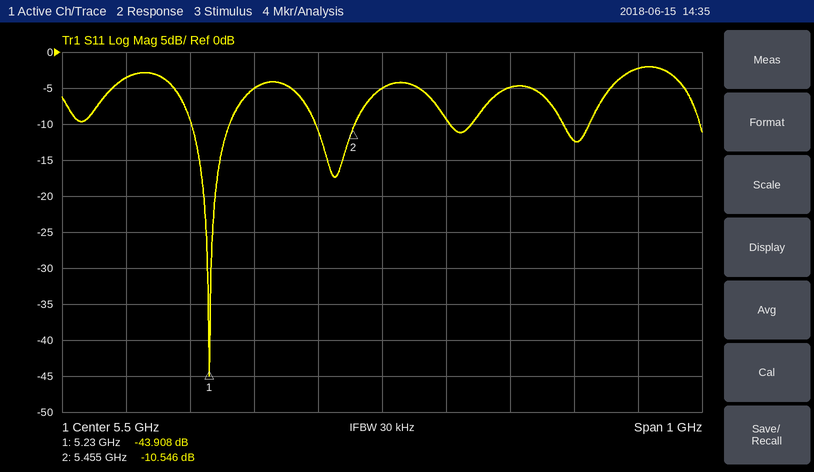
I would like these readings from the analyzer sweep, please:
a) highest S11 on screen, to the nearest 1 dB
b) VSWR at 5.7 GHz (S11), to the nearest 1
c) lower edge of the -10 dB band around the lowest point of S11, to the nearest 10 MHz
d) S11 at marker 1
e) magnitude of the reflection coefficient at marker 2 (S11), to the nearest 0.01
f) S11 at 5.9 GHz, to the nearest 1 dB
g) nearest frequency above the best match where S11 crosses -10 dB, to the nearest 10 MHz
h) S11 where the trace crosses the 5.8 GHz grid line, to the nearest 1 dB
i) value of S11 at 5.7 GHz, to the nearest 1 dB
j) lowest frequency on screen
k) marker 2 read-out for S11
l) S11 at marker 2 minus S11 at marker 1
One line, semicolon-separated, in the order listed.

-2 dB; 4; 5.20 GHz; -43.908 dB; 0.30; -2 dB; 5.26 GHz; -12 dB; -5 dB; 5 GHz; -10.546 dB; 33.362 dB
